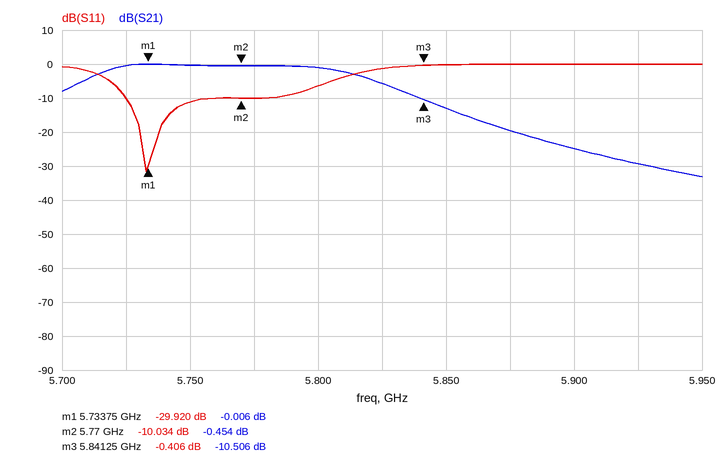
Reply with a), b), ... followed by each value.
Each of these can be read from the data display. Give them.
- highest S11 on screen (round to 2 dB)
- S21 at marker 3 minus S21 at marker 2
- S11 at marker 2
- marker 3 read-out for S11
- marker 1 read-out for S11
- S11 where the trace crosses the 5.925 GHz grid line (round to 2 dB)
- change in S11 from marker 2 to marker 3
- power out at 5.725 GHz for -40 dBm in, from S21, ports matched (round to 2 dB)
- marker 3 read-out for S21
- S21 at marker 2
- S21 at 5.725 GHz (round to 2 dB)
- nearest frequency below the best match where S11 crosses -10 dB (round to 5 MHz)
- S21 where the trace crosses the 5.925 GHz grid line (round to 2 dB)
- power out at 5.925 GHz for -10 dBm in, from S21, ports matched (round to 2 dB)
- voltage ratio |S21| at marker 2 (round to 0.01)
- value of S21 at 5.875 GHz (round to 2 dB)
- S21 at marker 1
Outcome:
a) 0 dB
b) -10.052 dB
c) -10.034 dB
d) -0.406 dB
e) -29.920 dB
f) 0 dB
g) 9.628 dB
h) -40 dBm
i) -10.506 dB
j) -0.454 dB
k) 0 dB
l) 5.725 GHz
m) -30 dB
n) -40 dBm
o) 0.95
p) -20 dB
q) -0.006 dB
